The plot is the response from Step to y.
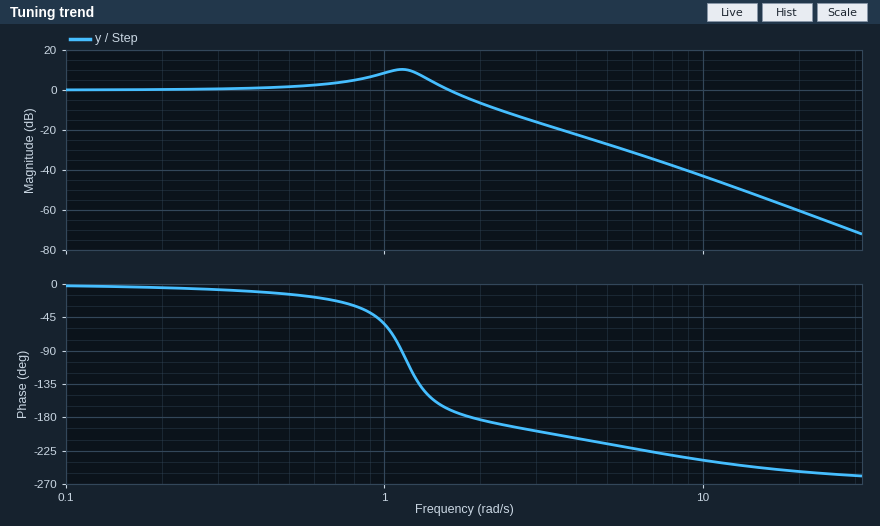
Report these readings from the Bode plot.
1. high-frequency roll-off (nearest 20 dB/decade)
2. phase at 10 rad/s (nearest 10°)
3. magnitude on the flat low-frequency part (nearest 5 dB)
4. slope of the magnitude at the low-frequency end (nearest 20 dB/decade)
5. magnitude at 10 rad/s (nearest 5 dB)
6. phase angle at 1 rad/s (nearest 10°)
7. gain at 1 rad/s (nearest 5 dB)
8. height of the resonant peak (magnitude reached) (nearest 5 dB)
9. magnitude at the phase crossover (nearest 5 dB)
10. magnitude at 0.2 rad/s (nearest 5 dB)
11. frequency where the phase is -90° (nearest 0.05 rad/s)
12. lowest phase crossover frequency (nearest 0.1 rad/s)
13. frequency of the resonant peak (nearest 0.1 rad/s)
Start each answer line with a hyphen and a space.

- -60 dB/decade
- -240°
- 0 dB
- 0 dB/decade
- -45 dB
- -50°
- 10 dB
- 10 dB
- -5 dB
- 0 dB
- 1.15 rad/s
- 1.9 rad/s
- 1.1 rad/s
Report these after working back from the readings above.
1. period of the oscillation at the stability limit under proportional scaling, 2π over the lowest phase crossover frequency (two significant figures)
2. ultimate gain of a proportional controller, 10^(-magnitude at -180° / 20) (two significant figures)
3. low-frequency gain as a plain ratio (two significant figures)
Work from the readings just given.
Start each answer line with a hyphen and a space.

- 3.3 s
- 1.8
- 1.0
